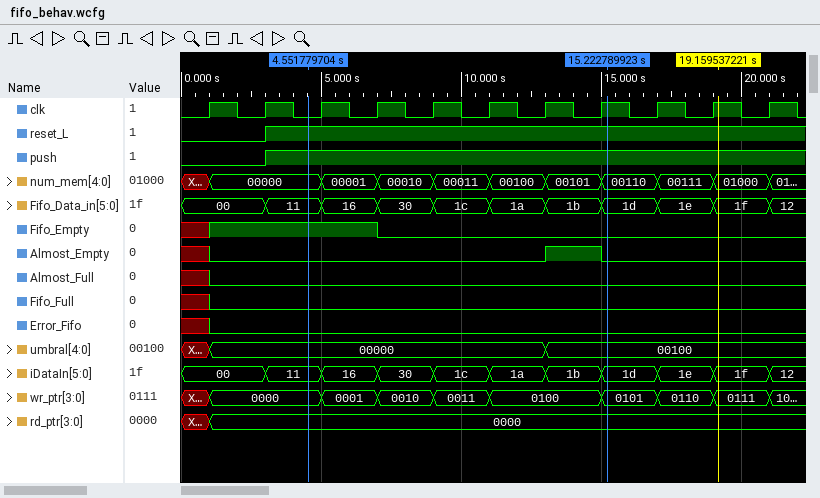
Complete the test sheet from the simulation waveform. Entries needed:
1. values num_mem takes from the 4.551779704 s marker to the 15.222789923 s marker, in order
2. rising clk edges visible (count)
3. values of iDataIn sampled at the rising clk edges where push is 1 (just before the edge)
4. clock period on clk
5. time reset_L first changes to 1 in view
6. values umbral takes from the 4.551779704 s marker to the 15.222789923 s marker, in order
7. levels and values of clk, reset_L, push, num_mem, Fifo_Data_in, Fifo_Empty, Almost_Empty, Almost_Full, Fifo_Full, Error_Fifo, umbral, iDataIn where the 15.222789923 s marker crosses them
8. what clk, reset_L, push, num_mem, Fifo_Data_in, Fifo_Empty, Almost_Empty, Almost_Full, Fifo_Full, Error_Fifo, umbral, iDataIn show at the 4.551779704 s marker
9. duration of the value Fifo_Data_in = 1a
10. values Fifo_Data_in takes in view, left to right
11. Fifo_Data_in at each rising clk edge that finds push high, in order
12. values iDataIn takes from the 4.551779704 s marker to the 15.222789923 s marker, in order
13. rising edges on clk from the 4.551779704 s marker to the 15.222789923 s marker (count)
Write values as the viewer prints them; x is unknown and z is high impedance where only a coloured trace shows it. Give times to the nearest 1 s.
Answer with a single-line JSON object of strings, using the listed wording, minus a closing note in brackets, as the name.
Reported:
{"values num_mem takes from the 4.551779704 s marker to the 15.222789923 s marker, in order": "00000, 00001, 00010, 00011, 00100, 00101, 00110", "rising clk edges visible": "11", "values of iDataIn sampled at the rising clk edges where push is 1": "11, 16, 30, 1c, 1a, 1b, 1d, 1e, 1f", "clock period on clk": "2 s", "time reset_L first changes to 1 in view": "3 s", "values umbral takes from the 4.551779704 s marker to the 15.222789923 s marker, in order": "00000, 00100", "levels and values of clk, reset_L, push, num_mem, Fifo_Data_in, Fifo_Empty, Almost_Empty, Almost_Full, Fifo_Full, Error_Fifo, umbral, iDataIn where the 15.222789923 s marker crosses them": "clk=1, reset_L=1, push=1, num_mem=00110, Fifo_Data_in=1d, Fifo_Empty=0, Almost_Empty=0, Almost_Full=0, Fifo_Full=0, Error_Fifo=0, umbral=00100, iDataIn=1d", "what clk, reset_L, push, num_mem, Fifo_Data_in, Fifo_Empty, Almost_Empty, Almost_Full, Fifo_Full, Error_Fifo, umbral, iDataIn show at the 4.551779704 s marker": "clk=0, reset_L=1, push=1, num_mem=00000, Fifo_Data_in=11, Fifo_Empty=1, Almost_Empty=0, Almost_Full=0, Fifo_Full=0, Error_Fifo=0, umbral=00000, iDataIn=11", "duration of the value Fifo_Data_in = 1a": "2 s", "values Fifo_Data_in takes in view, left to right": "00, 11, 16, 30, 1c, 1a, 1b, 1d, 1e, 1f, 12", "Fifo_Data_in at each rising clk edge that finds push high, in order": "11, 16, 30, 1c, 1a, 1b, 1d, 1e, 1f", "values iDataIn takes from the 4.551779704 s marker to the 15.222789923 s marker, in order": "11, 16, 30, 1c, 1a, 1b, 1d", "rising edges on clk from the 4.551779704 s marker to the 15.222789923 s marker": "6"}
